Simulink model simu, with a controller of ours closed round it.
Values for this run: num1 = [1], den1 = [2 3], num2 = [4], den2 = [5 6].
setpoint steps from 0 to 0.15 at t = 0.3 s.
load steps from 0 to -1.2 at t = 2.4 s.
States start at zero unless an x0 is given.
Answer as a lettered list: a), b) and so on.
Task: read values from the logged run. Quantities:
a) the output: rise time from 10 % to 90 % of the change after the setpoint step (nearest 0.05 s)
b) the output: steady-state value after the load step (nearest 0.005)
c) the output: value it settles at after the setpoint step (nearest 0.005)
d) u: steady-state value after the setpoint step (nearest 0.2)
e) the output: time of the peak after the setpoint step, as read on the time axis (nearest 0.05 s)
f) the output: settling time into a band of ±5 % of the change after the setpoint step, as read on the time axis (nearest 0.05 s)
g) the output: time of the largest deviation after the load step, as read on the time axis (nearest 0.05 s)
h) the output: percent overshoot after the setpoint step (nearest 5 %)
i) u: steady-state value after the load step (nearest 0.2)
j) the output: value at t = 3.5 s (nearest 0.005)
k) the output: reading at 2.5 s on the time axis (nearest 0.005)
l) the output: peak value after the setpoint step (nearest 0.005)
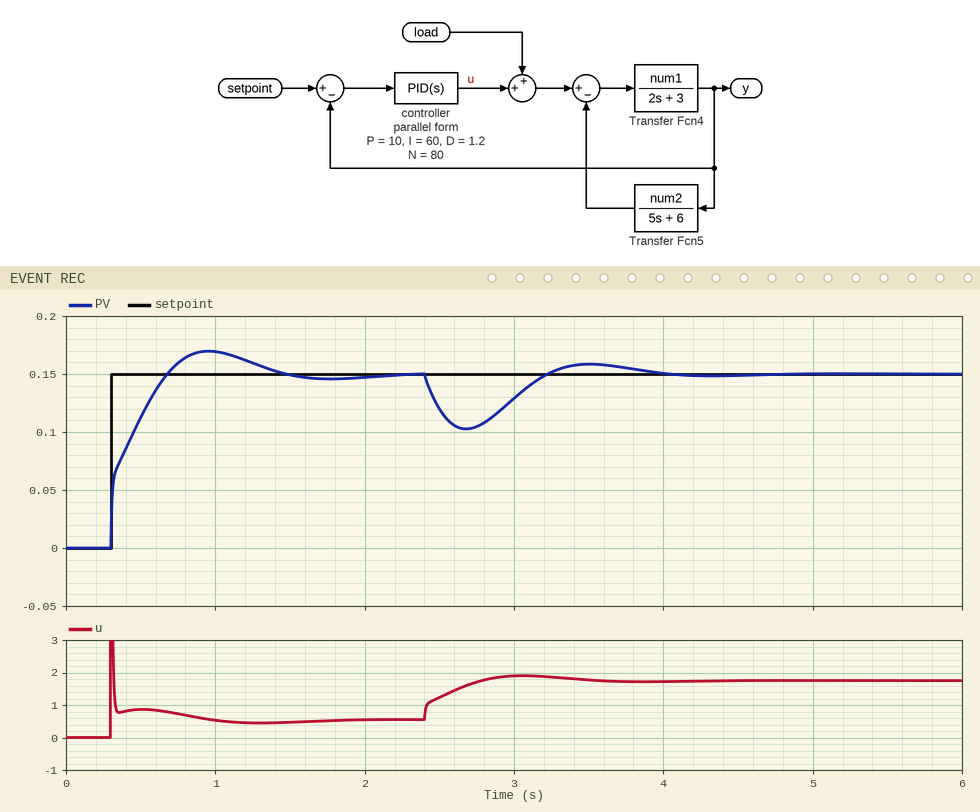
a) 0.30 s
b) 0.150
c) 0.150
d) 0.6
e) 0.95 s
f) 1.30 s
g) 2.70 s
h) 15 %
i) 1.8
j) 0.160
k) 0.120
l) 0.170
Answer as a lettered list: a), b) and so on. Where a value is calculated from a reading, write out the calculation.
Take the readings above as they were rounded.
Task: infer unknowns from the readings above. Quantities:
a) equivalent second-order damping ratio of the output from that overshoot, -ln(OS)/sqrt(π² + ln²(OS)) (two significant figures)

a) ln(0.15) = -1.897; 1.897 / sqrt(9.870 + 3.599) = 0.52
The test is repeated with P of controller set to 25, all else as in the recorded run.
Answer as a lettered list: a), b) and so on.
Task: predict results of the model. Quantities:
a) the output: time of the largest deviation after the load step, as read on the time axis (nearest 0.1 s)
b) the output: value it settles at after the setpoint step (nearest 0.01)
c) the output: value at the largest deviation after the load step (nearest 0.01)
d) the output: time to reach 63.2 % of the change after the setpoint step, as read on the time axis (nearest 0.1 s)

a) 2.6 s
b) 0.15
c) 0.12
d) 0.4 s
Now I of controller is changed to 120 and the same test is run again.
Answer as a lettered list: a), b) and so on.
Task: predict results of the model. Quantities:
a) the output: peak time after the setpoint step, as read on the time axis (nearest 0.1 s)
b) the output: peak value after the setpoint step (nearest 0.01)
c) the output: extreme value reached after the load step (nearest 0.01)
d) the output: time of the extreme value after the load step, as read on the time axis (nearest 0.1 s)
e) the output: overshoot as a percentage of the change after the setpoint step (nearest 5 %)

a) 0.8 s
b) 0.18
c) 0.11
d) 2.6 s
e) 20 %
